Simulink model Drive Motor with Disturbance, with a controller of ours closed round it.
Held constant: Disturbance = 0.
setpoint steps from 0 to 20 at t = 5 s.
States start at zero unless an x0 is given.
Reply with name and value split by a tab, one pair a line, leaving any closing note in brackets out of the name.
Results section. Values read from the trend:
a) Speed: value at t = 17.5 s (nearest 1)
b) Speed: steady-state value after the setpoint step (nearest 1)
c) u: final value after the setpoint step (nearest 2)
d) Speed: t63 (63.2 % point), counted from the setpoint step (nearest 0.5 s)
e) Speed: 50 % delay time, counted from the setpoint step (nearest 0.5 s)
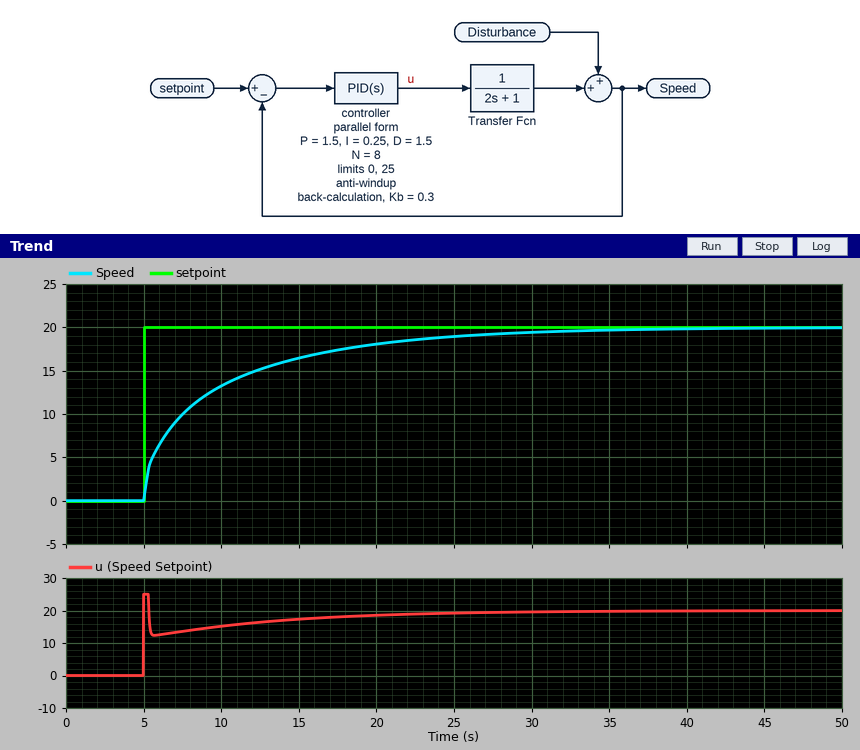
Speed: value at t = 17.5 s	17
Speed: steady-state value after the setpoint step	20
u: final value after the setpoint step	20
Speed: t63 (63.2 % point), counted from the setpoint step	4.5 s
Speed: 50 % delay time, counted from the setpoint step	2.5 s
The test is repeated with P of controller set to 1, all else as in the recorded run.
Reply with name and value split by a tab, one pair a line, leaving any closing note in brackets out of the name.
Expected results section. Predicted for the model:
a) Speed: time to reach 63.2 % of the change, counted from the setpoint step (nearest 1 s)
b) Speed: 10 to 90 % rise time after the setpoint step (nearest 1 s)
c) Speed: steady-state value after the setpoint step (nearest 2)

Speed: time to reach 63.2 % of the change, counted from the setpoint step	5 s
Speed: 10 to 90 % rise time after the setpoint step	13 s
Speed: steady-state value after the setpoint step	20
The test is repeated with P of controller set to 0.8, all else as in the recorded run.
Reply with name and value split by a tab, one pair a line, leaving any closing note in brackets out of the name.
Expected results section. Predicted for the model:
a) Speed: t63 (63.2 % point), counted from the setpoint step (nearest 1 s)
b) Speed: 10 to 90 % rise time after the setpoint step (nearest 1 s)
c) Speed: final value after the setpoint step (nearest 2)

Speed: t63 (63.2 % point), counted from the setpoint step	6 s
Speed: 10 to 90 % rise time after the setpoint step	12 s
Speed: final value after the setpoint step	20
